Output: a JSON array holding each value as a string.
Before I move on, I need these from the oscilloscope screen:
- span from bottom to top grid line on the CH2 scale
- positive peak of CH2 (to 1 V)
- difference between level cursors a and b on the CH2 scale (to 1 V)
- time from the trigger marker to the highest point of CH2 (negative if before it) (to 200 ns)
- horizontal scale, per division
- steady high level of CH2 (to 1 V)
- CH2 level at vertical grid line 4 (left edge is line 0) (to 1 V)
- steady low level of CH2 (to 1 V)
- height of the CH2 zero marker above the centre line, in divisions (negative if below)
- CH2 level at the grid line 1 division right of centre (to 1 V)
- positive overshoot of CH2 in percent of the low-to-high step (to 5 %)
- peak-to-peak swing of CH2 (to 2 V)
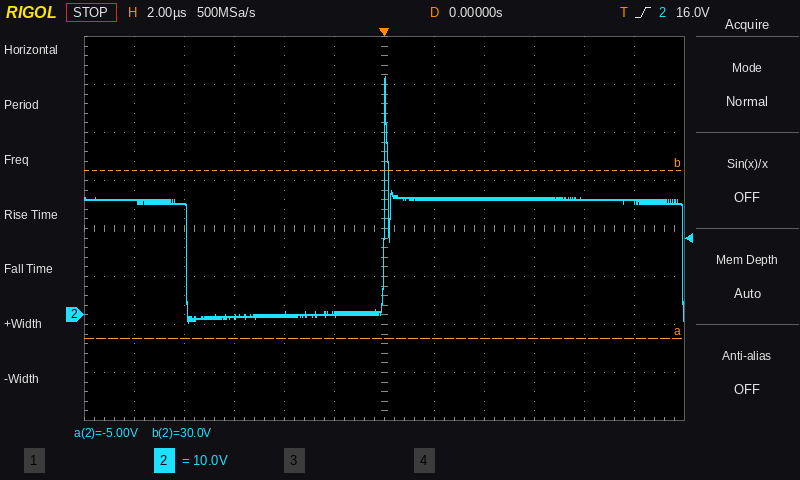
["80 V", "50 V", "35 V", "0.0 µs", "2 µs", "24 V", "0 V", "0 V", "-1.8 div", "24 V", "105 %", "52 V"]
